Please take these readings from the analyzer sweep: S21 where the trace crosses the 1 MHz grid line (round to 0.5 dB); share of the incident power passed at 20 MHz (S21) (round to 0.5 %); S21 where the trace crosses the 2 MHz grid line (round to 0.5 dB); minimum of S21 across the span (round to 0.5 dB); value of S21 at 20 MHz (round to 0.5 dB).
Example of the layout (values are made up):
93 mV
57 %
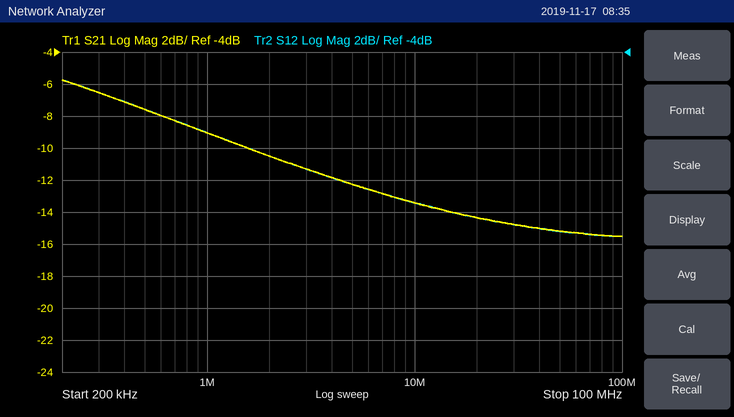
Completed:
-9.0 dB
3.5 %
-10.5 dB
-15.5 dB
-14.5 dB
